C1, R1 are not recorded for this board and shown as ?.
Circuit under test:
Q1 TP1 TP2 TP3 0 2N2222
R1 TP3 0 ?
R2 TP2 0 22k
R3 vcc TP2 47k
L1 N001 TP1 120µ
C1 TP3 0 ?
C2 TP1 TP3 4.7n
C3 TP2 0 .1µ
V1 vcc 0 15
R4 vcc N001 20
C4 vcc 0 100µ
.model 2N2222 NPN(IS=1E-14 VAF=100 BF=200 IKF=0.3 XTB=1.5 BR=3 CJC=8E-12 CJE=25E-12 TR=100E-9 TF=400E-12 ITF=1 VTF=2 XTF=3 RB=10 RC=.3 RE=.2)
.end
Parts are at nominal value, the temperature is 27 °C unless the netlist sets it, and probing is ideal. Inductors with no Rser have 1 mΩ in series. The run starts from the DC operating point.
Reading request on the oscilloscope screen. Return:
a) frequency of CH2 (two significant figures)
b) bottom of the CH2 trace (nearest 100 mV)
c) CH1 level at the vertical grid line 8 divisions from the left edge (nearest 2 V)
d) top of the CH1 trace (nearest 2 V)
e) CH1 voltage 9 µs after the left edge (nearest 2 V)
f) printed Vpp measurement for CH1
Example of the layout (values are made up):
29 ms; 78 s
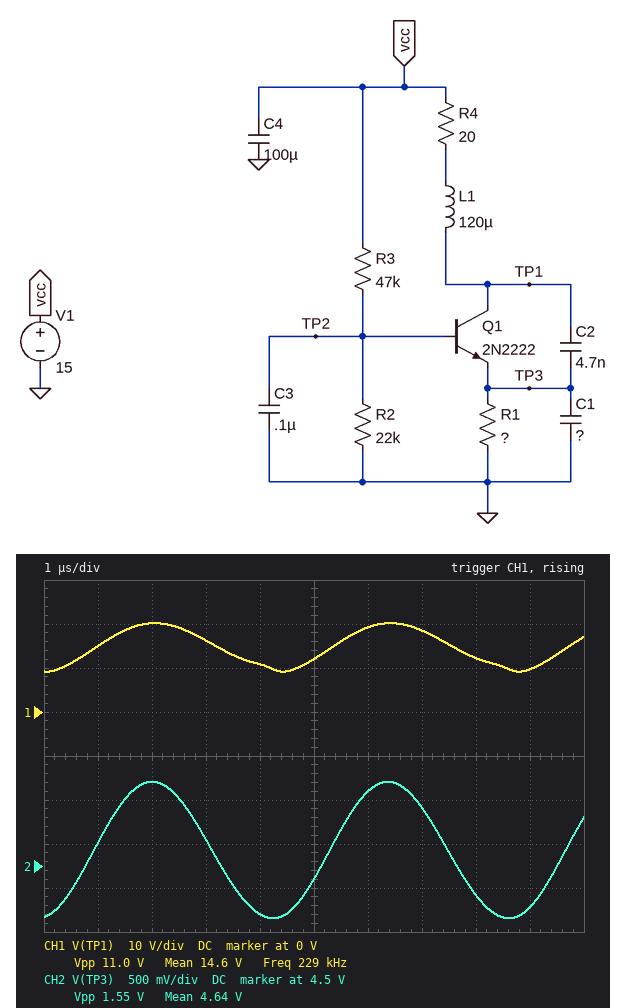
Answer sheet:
230 kHz; 3.9 V; 12 V; 20 V; 10 V; 11.0 V
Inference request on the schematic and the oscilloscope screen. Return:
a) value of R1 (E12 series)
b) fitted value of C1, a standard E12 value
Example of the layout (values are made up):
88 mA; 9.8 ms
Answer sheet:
2.2 kΩ; 27 nF
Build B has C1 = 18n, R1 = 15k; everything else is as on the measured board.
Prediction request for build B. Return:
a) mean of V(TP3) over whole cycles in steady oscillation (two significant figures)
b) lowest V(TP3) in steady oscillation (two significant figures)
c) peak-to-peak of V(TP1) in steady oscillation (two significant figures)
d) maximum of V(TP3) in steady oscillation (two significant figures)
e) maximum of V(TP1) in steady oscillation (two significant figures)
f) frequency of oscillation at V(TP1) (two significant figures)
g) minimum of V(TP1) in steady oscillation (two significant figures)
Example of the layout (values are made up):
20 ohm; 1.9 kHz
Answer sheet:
4.2 V; 4.1 V; 1.3 V; 4.4 V; 16 V; 240 kHz; 14 V
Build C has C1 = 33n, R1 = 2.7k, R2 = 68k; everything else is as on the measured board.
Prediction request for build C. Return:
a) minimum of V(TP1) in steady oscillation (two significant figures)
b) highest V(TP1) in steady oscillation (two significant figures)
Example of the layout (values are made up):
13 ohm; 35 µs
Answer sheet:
7.4 V; 22 V
